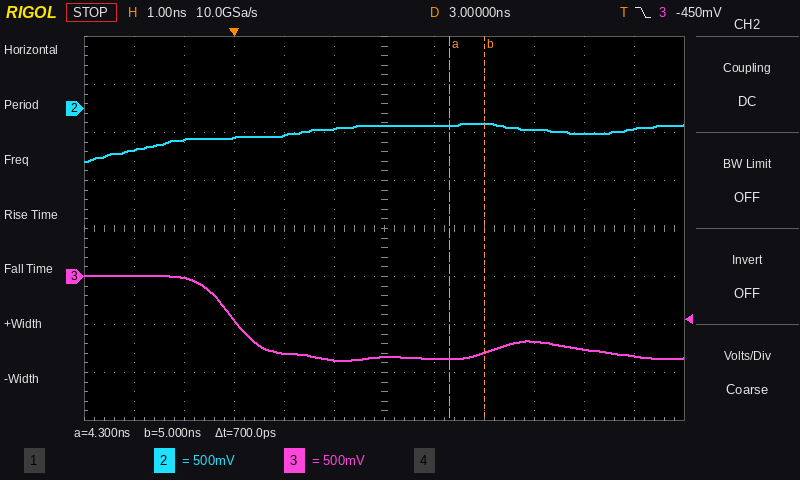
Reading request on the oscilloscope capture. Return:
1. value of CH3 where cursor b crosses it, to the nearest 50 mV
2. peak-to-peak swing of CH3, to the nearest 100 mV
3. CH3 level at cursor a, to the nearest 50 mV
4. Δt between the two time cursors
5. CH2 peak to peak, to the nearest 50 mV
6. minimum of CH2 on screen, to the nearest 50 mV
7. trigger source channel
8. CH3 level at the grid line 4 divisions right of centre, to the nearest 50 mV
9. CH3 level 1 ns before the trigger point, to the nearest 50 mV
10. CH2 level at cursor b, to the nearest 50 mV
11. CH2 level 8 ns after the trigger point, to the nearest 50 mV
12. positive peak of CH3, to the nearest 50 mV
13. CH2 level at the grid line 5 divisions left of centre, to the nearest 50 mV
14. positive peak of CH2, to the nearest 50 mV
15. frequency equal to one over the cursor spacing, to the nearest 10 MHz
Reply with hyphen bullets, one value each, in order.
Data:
- -800 mV
- 900 mV
- -850 mV
- 700 ps
- 400 mV
- -550 mV
- CH3
- -750 mV
- 0 mV
- -150 mV
- -200 mV
- 0 mV
- -450 mV
- -150 mV
- 1.43 GHz
